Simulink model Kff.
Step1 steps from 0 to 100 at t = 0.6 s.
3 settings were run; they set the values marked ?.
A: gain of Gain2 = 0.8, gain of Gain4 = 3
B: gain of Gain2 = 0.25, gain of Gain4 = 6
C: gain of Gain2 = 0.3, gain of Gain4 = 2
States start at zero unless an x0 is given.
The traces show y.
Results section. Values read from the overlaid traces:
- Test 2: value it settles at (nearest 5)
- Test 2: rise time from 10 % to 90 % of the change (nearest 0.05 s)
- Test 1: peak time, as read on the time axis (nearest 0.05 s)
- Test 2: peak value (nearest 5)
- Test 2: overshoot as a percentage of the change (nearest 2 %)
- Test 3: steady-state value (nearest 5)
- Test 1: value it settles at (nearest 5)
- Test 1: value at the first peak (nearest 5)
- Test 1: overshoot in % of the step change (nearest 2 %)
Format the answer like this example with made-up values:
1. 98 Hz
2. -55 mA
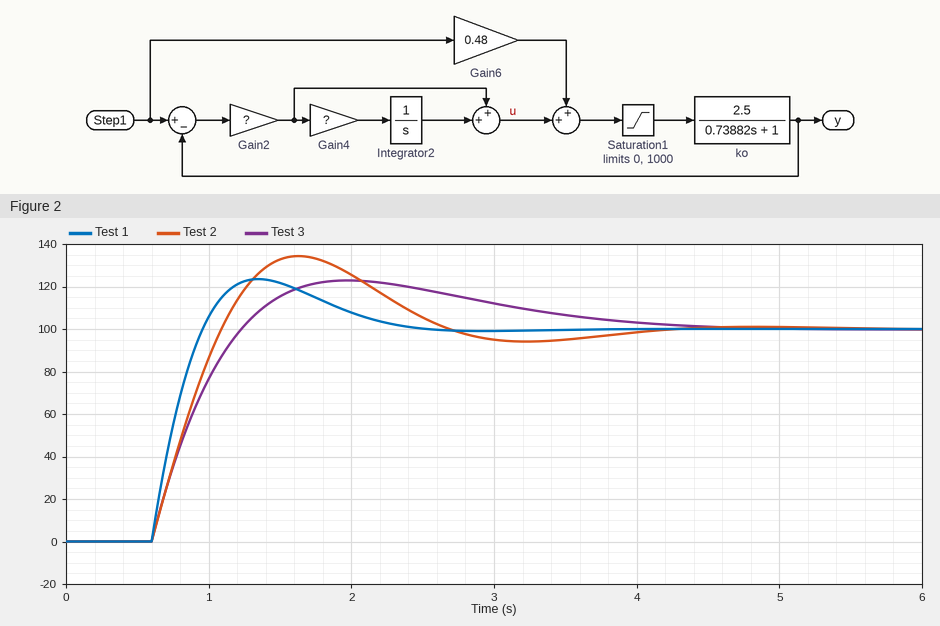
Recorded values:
1. 100
2. 0.40 s
3. 1.35 s
4. 135
5. 34 %
6. 100
7. 100
8. 125
9. 24 %
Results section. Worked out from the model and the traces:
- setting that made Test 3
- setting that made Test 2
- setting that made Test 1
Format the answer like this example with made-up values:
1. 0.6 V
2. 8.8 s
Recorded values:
1. C
2. B
3. A
